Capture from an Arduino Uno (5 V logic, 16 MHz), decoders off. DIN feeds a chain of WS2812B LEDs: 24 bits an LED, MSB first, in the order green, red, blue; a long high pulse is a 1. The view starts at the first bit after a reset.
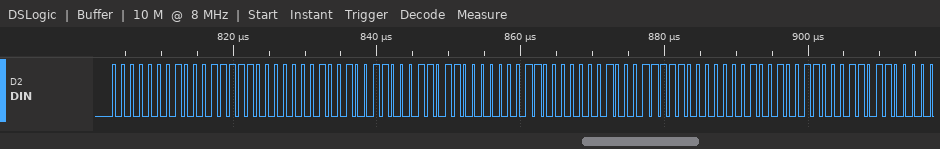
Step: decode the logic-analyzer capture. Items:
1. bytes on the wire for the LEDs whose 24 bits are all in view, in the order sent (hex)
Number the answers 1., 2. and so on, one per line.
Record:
1. 01 1F 01 26 36 03 01 1F 01
